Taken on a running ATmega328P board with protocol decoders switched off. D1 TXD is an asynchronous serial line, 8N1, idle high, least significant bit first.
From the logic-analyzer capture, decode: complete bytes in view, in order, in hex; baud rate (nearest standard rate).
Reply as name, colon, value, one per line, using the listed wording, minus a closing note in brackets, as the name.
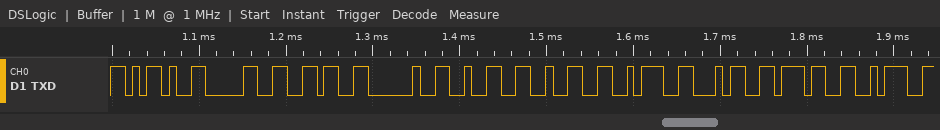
complete bytes in view, in order, in hex: 0x2D 0x30 0x36 0x20 0x32 0x32 0x3A 0x34 0x37 0x3A
baud rate: 115200 baud
